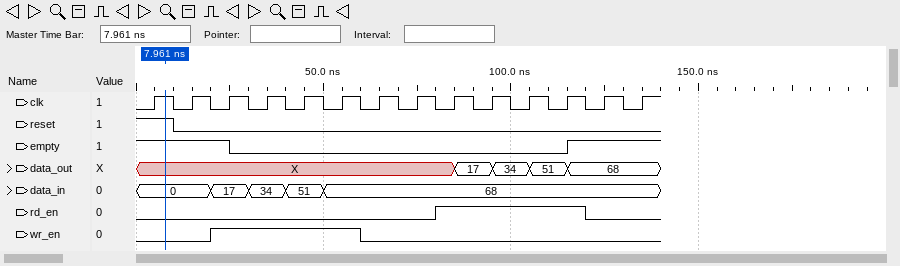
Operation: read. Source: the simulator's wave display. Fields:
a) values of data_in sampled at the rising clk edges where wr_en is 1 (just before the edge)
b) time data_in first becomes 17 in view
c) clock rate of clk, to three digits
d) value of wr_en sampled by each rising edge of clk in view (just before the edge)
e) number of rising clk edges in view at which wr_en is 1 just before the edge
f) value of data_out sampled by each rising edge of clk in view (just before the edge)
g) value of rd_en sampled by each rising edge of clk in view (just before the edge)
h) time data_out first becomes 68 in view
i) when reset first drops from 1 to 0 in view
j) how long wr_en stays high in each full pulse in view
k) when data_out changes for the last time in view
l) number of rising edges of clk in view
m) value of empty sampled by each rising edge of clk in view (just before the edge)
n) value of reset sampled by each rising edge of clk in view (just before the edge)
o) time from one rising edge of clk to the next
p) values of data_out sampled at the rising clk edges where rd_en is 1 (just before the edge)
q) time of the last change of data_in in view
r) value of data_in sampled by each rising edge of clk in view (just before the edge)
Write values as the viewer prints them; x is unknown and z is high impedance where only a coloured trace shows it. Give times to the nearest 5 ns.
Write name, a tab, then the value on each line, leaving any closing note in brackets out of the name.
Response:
values of data_in sampled at the rising clk edges where wr_en is 1	17, 34, 51, 68
time data_in first becomes 17 in view	20 ns
clock rate of clk, to three digits	100 MHz
value of wr_en sampled by each rising edge of clk in view	0 0 1 1 1 1 0 0 0 0 0 0 0 0
number of rising clk edges in view at which wr_en is 1 just before the edge	4
value of data_out sampled by each rising edge of clk in view	X, X, X, X, X, X, X, X, X, 17, 34, 51, 68, 68
value of rd_en sampled by each rising edge of clk in view	0 0 0 0 0 0 0 0 1 1 1 1 0 0
time data_out first becomes 68 in view	115 ns
when reset first drops from 1 to 0 in view	10 ns
how long wr_en stays high in each full pulse in view	40 ns
when data_out changes for the last time in view	115 ns
number of rising edges of clk in view	14
value of empty sampled by each rising edge of clk in view	1 1 1 0 0 0 0 0 0 0 0 0 1 1
value of reset sampled by each rising edge of clk in view	1 0 0 0 0 0 0 0 0 0 0 0 0 0
time from one rising edge of clk to the next	10 ns
values of data_out sampled at the rising clk edges where rd_en is 1	X, 17, 34, 51
time of the last change of data_in in view	50 ns
value of data_in sampled by each rising edge of clk in view	0, 0, 17, 34, 51, 68, 68, 68, 68, 68, 68, 68, 68, 68
